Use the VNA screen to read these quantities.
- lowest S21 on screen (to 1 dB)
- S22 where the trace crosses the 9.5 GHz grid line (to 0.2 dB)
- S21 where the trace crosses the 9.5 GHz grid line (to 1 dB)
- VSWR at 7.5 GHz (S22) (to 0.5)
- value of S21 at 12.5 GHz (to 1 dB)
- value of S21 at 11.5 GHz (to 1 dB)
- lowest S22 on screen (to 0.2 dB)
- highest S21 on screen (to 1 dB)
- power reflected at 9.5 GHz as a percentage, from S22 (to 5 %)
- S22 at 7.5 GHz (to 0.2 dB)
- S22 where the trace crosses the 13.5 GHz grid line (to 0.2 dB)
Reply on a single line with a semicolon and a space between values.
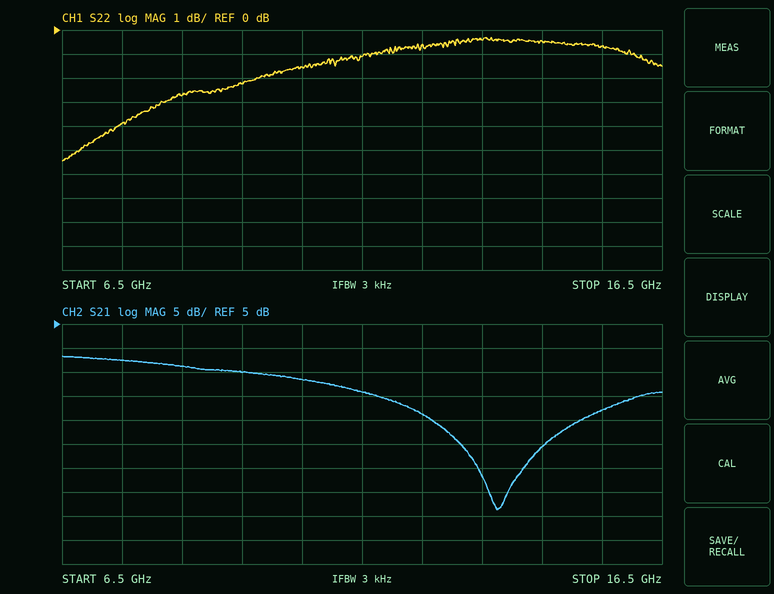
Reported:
-34 dB; -2.2 dB; -5 dB; 4.5; -14 dB; -9 dB; -5.4 dB; -2 dB; 60 %; -3.8 dB; -0.4 dB
